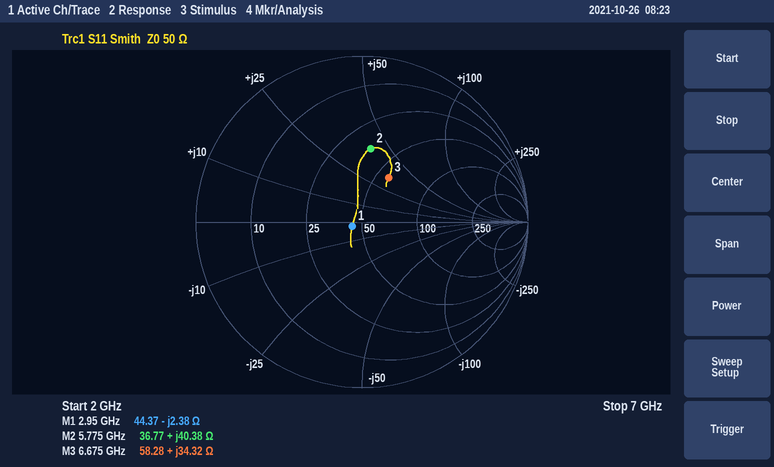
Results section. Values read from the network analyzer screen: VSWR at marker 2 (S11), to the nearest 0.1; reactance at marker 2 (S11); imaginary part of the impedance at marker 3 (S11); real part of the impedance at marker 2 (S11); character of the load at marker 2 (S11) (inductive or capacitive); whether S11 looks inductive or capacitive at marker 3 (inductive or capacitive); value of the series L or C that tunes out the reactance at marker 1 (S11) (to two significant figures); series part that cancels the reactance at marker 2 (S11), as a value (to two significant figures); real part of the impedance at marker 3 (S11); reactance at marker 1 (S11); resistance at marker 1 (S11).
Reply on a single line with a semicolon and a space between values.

2.6; +40.38 Ω; +34.32 Ω; 36.77 Ω; inductive; inductive; 130 pH; 680 fF; 58.28 Ω; -2.38 Ω; 44.37 Ω
